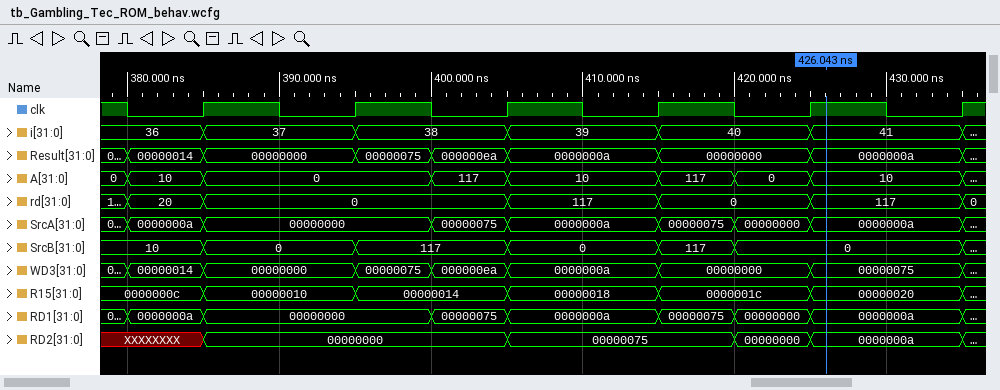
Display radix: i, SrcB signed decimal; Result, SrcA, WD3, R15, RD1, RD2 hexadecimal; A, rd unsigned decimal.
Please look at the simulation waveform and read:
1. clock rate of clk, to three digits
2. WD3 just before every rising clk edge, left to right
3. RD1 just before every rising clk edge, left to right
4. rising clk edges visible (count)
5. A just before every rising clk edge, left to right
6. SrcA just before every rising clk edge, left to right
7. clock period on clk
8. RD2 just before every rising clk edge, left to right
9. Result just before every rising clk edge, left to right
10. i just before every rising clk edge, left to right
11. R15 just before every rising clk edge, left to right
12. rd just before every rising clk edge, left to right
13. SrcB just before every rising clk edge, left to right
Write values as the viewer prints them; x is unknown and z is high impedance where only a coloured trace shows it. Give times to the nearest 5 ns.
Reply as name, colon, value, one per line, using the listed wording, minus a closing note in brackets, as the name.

clock rate of clk, to three digits: 100 MHz
WD3 just before every rising clk edge, left to right: 00000014, 00000000, 000000ea, 0000000a, 00000000, 00000075
RD1 just before every rising clk edge, left to right: 0000000a, 00000000, 00000075, 0000000a, 00000000, 0000000a
rising clk edges visible: 6
A just before every rising clk edge, left to right: 10, 0, 117, 10, 0, 10
SrcA just before every rising clk edge, left to right: 0000000a, 00000000, 00000075, 0000000a, 00000000, 0000000a
clock period on clk: 10 ns
RD2 just before every rising clk edge, left to right: XXXXXXXX, 00000000, 00000000, 00000075, 00000000, 0000000a
Result just before every rising clk edge, left to right: 00000014, 00000000, 000000ea, 0000000a, 00000000, 0000000a
i just before every rising clk edge, left to right: 36, 37, 38, 39, 40, 41
R15 just before every rising clk edge, left to right: 0000000c, 00000010, 00000014, 00000018, 0000001c, 00000020
rd just before every rising clk edge, left to right: 20, 0, 0, 117, 0, 117
SrcB just before every rising clk edge, left to right: 10, 0, 117, 0, 0, 0
